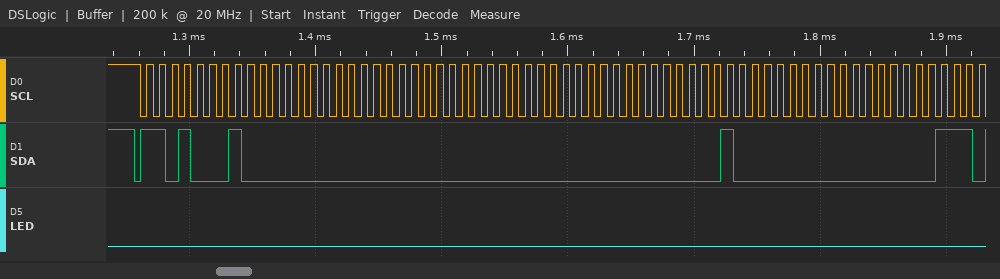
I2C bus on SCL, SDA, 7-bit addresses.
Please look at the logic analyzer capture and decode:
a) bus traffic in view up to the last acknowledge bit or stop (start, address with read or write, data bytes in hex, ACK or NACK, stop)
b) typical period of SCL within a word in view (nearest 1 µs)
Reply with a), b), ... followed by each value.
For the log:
a) start, address 68 read ACK, 00 ACK, 00 ACK, 00 ACK, 00 ACK, 40 ACK, 00 ACK
b) 10 µs
